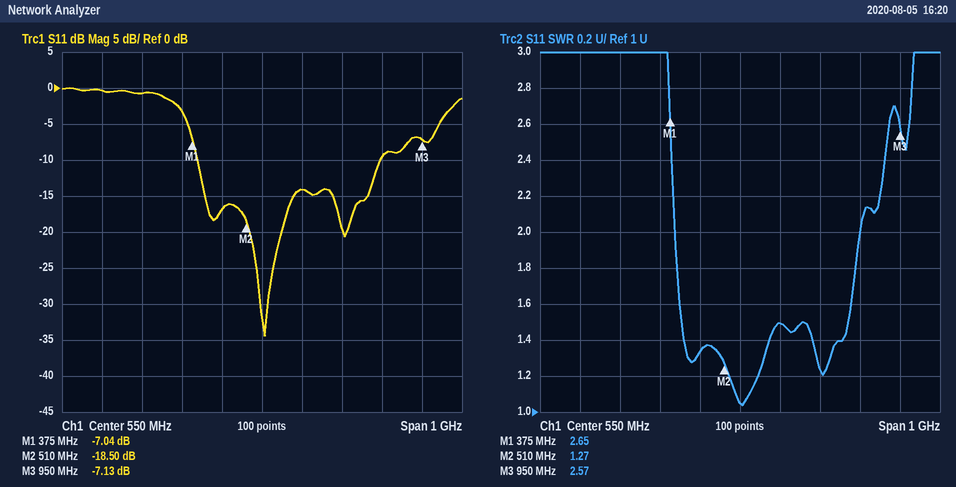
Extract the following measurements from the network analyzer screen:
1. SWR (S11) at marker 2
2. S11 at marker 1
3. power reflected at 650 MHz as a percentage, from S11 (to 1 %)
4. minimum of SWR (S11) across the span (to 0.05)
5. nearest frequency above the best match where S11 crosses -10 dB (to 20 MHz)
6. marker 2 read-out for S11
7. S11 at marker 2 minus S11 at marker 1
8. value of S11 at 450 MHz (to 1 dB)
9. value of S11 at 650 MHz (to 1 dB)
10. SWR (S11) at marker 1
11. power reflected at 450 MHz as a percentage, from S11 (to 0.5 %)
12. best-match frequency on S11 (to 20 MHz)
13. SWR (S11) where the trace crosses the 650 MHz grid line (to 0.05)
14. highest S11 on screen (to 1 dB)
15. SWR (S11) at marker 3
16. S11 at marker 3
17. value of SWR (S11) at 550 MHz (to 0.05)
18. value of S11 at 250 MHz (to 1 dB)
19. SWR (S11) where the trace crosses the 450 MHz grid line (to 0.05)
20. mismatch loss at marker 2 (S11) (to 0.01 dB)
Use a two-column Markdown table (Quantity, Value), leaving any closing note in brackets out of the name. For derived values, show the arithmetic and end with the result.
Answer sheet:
| Quantity | Value |
|---|---|
| SWR (S11) at marker 2 | 1.27 |
| S11 at marker 1 | -7.04 dB |
| power reflected at 650 MHz as a percentage, from S11 | 10^(-14/10) ≈ 4 % |
| minimum of SWR (S11) across the span | 1.05 |
| nearest frequency above the best match where S11 crosses -10 dB | 840 MHz |
| marker 2 read-out for S11 | -18.50 dB |
| S11 at marker 2 minus S11 at marker 1 | -18.5 − (-7.04) = -11.46 dB |
| value of S11 at 450 MHz | -17 dB |
| value of S11 at 650 MHz | -14 dB |
| SWR (S11) at marker 1 | 2.65 |
| power reflected at 450 MHz as a percentage, from S11 | 10^(-17/10) ≈ 2.0 % |
| best-match frequency on S11 | 560 MHz |
| SWR (S11) where the trace crosses the 650 MHz grid line | 1.50 |
| highest S11 on screen | 0 dB |
| SWR (S11) at marker 3 | 2.57 |
| S11 at marker 3 | -7.13 dB |
| value of SWR (S11) at 550 MHz | 1.05 |
| value of S11 at 250 MHz | -1 dB |
| SWR (S11) where the trace crosses the 450 MHz grid line | 1.35 |
| mismatch loss at marker 2 (S11) | −10 log10(1 − 10^(-18.5/10)) ≈ 0.06 dB |
